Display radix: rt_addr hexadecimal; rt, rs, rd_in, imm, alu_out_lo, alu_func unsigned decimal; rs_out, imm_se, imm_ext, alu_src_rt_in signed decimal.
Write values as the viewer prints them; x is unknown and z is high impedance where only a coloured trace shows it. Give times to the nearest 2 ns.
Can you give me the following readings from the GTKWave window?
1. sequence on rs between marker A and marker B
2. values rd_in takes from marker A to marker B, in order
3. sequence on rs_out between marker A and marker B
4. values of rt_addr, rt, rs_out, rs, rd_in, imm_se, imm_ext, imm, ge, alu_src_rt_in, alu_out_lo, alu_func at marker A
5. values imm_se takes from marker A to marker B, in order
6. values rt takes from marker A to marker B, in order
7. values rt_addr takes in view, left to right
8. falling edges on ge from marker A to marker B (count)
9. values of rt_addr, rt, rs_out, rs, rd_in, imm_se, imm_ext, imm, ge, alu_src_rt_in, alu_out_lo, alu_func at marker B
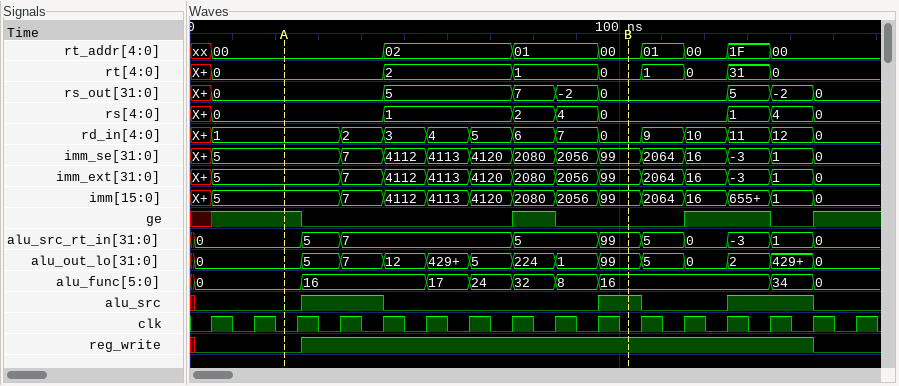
0, 1, 2, 4, 0
1, 2, 3, 4, 5, 6, 7, 0
0, 5, 7, -2, 0
rt_addr=00, rt=0, rs_out=0, rs=0, rd_in=1, imm_se=5, imm_ext=5, imm=5, ge=1, alu_src_rt_in=0, alu_out_lo=0, alu_func=0
5, 7, 4112, 4113, 4120, 2080, 2056, 99
0, 2, 1, 0
xx, 00, 02, 01, 00, 01, 00, 1F, 00
2
rt_addr=00, rt=0, rs_out=0, rs=0, rd_in=0, imm_se=99, imm_ext=99, imm=99, ge=0, alu_src_rt_in=99, alu_out_lo=99, alu_func=16
